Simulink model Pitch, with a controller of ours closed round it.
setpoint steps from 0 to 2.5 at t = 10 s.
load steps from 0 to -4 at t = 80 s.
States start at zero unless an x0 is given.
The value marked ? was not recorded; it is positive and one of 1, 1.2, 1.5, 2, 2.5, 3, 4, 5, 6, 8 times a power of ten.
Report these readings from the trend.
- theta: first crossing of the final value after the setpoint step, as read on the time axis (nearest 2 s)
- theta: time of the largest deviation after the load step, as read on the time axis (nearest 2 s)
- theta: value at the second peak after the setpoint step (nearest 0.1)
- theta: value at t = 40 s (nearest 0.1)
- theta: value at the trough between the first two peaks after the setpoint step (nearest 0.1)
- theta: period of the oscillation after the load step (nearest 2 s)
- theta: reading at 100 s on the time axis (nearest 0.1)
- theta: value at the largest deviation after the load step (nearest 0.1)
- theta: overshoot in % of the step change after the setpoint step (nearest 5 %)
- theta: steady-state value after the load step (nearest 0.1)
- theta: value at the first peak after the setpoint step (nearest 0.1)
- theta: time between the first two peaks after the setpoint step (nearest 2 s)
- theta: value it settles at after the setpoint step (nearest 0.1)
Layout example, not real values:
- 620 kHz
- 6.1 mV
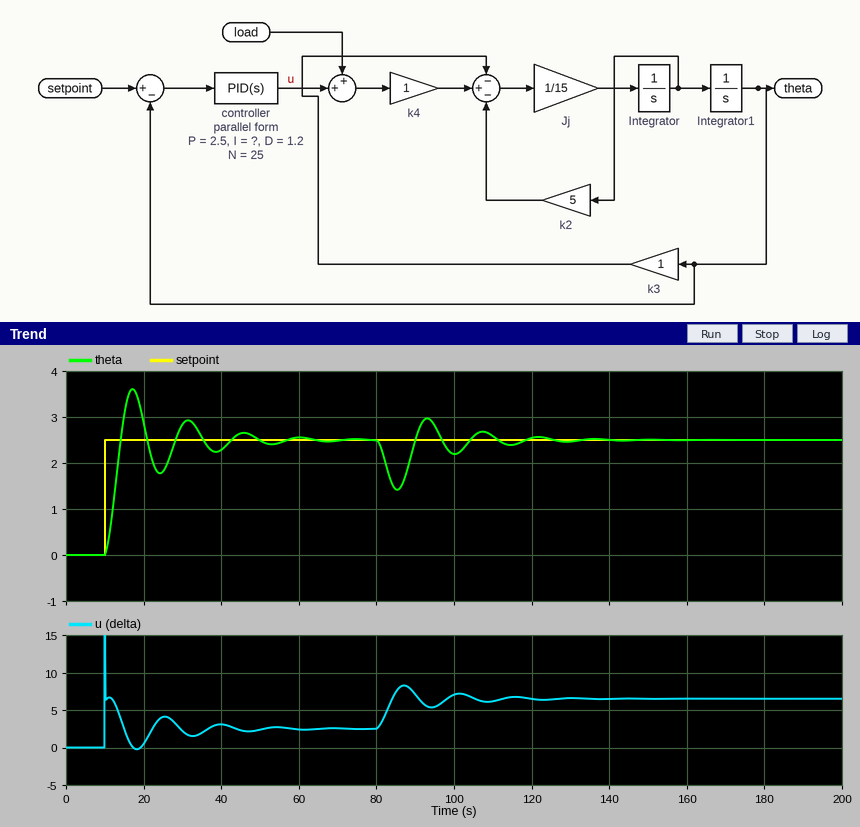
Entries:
- 14 s
- 86 s
- 2.9
- 2.3
- 1.8
- 14 s
- 2.2
- 1.4
- 45 %
- 2.5
- 3.6
- 14 s
- 2.5
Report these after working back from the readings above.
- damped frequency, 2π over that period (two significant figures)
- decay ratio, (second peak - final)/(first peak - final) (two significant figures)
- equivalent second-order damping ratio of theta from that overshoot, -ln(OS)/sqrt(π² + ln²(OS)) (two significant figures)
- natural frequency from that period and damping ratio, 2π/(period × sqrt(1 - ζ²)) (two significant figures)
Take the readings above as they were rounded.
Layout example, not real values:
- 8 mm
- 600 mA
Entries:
- 0.45 rad/s
- 0.36
- 0.25
- 0.46 rad/s
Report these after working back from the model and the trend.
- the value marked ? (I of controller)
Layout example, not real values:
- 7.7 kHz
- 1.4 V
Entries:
- 0.8
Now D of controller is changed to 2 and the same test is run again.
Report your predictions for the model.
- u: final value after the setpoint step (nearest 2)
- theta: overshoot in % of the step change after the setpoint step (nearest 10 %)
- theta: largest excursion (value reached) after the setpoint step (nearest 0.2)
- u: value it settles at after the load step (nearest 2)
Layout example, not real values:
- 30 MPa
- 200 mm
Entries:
- 2
- 40 %
- 3.4
- 6
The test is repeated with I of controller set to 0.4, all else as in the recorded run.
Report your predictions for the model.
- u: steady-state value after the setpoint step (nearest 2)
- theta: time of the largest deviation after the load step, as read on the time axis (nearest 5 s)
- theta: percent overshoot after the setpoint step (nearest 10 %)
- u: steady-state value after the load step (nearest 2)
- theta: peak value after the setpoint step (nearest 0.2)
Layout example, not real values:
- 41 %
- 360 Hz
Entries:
- 2
- 85 s
- 20 %
- 6
- 3.0
